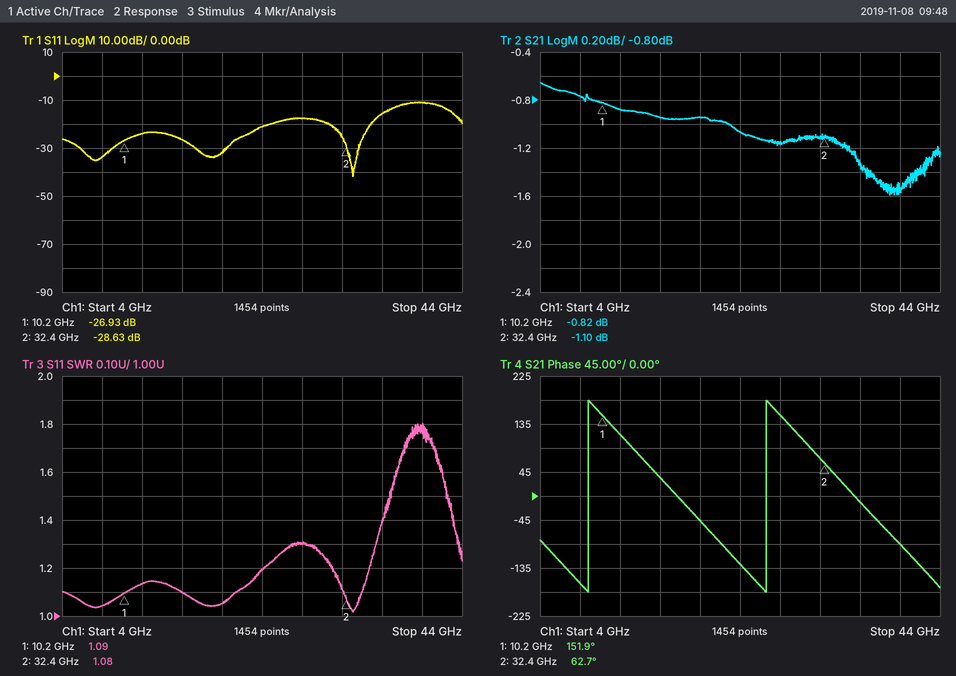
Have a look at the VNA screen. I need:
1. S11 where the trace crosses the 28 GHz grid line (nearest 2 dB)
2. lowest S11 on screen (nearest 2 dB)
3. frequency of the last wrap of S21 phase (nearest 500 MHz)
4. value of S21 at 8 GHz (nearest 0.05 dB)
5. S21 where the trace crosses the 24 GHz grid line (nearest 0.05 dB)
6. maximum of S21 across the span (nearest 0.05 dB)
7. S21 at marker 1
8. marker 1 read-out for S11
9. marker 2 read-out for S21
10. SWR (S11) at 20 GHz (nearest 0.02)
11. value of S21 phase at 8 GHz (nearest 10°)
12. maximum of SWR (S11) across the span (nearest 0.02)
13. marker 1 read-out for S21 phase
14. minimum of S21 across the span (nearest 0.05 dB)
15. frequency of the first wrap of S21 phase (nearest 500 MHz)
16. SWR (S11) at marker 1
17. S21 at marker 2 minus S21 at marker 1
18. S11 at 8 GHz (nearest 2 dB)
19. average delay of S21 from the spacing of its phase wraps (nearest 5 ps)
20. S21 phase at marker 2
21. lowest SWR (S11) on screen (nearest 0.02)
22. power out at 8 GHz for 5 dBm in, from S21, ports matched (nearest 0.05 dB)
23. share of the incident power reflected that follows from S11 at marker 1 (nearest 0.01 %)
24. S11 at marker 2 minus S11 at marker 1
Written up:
-18 dB
-42 dB
26.5 GHz
-0.75 dB
-1.05 dB
-0.65 dB
-0.82 dB
-26.93 dB
-1.10 dB
1.06
-160°
1.80
151.9°
-1.60 dB
9.0 GHz
1.09
-0.28 dB
-34 dB
55 ps
62.7°
1.02
4.25 dBm
0.20 %
-1.70 dB
